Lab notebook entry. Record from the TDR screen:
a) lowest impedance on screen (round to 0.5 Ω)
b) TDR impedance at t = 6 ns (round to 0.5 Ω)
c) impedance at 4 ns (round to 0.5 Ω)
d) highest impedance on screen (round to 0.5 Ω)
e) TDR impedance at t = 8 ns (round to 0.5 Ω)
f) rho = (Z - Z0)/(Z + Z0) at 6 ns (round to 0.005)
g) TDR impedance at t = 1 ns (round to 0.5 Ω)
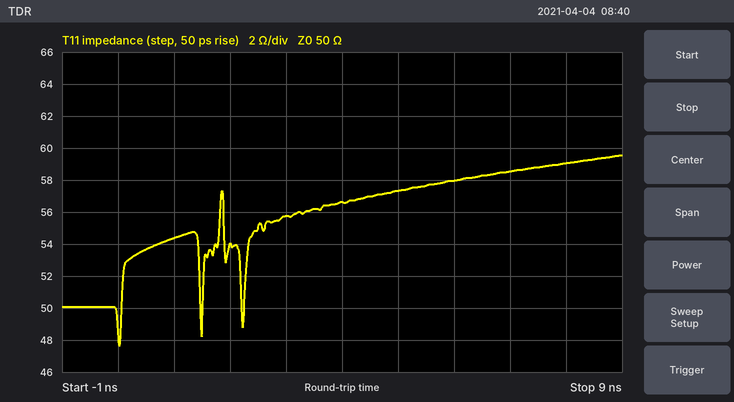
47.5 Ω
58.0 Ω
56.5 Ω
59.5 Ω
59.0 Ω
+0.075
54.5 Ω
